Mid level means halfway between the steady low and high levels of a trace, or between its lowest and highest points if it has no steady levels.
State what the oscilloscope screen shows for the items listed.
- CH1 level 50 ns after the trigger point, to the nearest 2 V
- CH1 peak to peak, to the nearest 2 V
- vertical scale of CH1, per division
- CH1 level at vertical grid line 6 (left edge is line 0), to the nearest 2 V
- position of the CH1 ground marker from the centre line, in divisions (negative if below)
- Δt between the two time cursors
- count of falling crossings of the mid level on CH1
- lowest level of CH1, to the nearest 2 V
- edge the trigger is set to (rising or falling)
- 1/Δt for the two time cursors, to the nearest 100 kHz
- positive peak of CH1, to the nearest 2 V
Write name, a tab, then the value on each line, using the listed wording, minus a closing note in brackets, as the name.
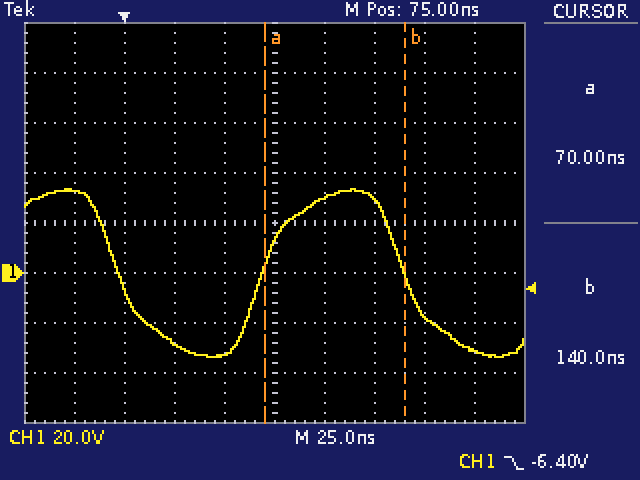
CH1 level 50 ns after the trigger point, to the nearest 2 V	-32 V
CH1 peak to peak, to the nearest 2 V	68 V
vertical scale of CH1, per division	20 V
CH1 level at vertical grid line 6 (left edge is line 0), to the nearest 2 V	30 V
position of the CH1 ground marker from the centre line, in divisions	-1.0 div
Δt between the two time cursors	70.0 ns
count of falling crossings of the mid level on CH1	2
lowest level of CH1, to the nearest 2 V	-34 V
edge the trigger is set to	falling
1/Δt for the two time cursors, to the nearest 100 kHz	14.3 MHz
positive peak of CH1, to the nearest 2 V	34 V
